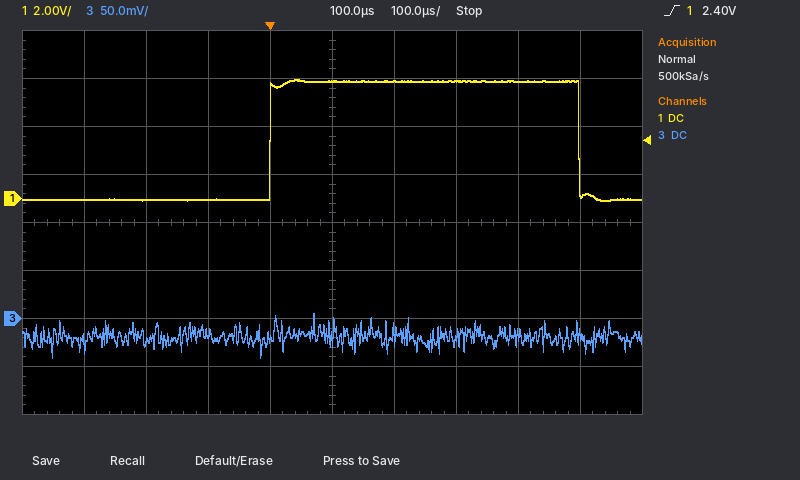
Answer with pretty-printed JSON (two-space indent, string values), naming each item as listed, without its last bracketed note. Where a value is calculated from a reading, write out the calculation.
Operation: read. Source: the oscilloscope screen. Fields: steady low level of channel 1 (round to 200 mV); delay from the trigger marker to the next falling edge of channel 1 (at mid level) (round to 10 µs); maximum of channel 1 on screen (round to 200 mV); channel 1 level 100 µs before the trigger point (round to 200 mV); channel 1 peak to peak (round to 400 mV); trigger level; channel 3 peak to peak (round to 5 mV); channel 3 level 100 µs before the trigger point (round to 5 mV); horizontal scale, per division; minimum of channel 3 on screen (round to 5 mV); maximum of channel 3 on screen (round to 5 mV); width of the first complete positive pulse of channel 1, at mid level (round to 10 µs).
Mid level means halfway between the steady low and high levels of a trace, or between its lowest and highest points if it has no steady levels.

{
  "steady low level of channel 1": "0.0 V",
  "delay from the trigger marker to the next falling edge of channel 1 (at mid level)": "500 µs",
  "maximum of channel 1 on screen": "5.0 V",
  "channel 1 level 100 µs before the trigger point": "0.0 V",
  "channel 1 peak to peak": "5.2 V",
  "trigger level": "2.40 V",
  "channel 3 peak to peak": "5 mV − (-40 mV) = 45 mV",
  "channel 3 level 100 µs before the trigger point": "-15 mV",
  "horizontal scale, per division": "100 µs",
  "minimum of channel 3 on screen": "-40 mV",
  "maximum of channel 3 on screen": "5 mV",
  "width of the first complete positive pulse of channel 1, at mid level": "500 µs"
}
